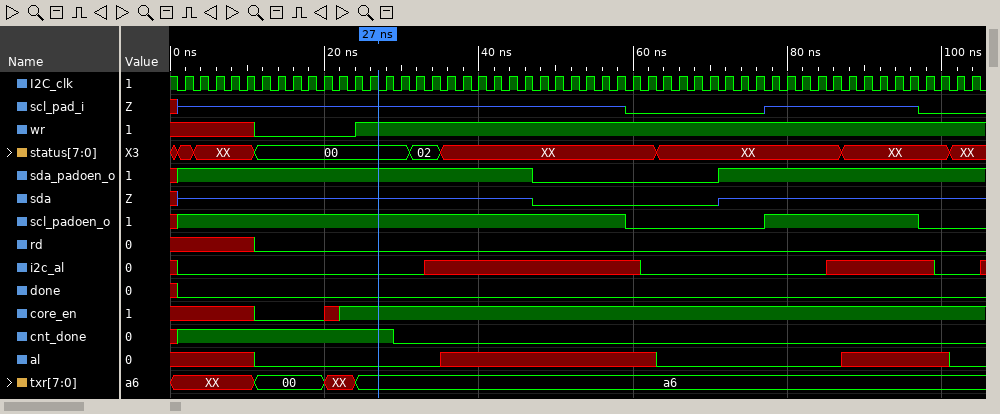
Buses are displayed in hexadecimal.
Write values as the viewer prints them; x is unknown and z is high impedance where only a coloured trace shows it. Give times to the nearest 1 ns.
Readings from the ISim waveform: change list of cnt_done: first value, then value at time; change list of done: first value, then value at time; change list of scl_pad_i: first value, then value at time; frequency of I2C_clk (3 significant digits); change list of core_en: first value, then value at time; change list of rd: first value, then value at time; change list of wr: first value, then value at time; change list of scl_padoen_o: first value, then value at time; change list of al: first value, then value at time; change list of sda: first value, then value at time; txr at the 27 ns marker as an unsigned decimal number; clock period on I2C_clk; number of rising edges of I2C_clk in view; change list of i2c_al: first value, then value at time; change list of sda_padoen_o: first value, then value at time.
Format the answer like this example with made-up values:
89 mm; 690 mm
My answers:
x, 1 at 1 ns, 0 at 29 ns; x, 0 at 1 ns; x, z at 1 ns, 0 at 59 ns, z at 77 ns, 0 at 97 ns; 500 MHz; x, 0 at 11 ns, x at 20 ns, 1 at 22 ns; x, 0 at 11 ns; x, 0 at 11 ns, 1 at 24 ns; x, 1 at 1 ns, 0 at 59 ns, 1 at 77 ns, 0 at 97 ns; x, 0 at 11 ns, x at 35 ns, 0 at 63 ns, x at 87 ns, 0 at 101 ns; x, z at 1 ns, 0 at 47 ns, z at 71 ns; 166; 2 ns; 52; x, 0 at 1 ns, x at 33 ns, 0 at 61 ns, x at 85 ns, 0 at 99 ns, x at 105 ns; x, 1 at 1 ns, 0 at 47 ns, 1 at 71 ns
